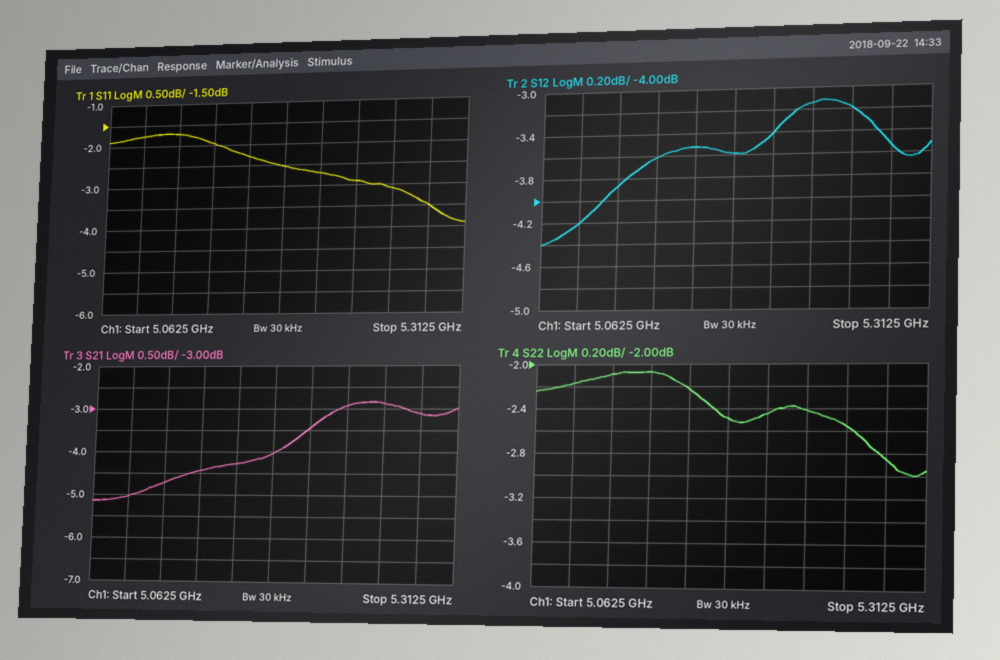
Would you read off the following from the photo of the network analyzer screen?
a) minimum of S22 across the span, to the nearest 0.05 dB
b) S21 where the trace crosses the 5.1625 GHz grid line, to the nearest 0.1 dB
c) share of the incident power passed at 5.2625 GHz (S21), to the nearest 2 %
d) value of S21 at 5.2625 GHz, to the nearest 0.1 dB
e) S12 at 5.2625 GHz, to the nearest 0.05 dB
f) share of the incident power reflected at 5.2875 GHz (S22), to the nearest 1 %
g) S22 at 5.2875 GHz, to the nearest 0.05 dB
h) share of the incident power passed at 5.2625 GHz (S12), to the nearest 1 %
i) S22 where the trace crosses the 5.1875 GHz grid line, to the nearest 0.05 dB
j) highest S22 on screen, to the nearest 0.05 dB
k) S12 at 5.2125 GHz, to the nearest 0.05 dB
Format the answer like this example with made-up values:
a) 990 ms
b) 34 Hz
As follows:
a) -3.00 dB
b) -4.3 dB
c) 52 %
d) -2.9 dB
e) -3.20 dB
f) 52 %
g) -2.85 dB
h) 48 %
i) -2.50 dB
j) -2.05 dB
k) -3.40 dB
